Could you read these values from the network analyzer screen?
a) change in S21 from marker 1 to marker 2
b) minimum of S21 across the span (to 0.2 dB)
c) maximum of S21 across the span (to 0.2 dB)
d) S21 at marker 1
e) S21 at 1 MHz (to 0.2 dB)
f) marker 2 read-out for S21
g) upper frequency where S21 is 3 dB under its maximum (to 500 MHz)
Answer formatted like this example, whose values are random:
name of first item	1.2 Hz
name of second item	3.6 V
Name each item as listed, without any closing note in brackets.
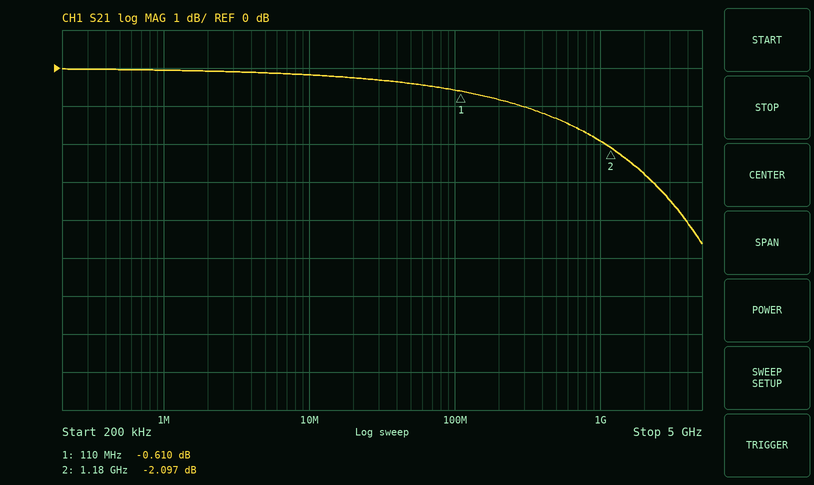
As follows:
change in S21 from marker 1 to marker 2	-1.487 dB
minimum of S21 across the span	-4.6 dB
maximum of S21 across the span	0.0 dB
S21 at marker 1	-0.610 dB
S21 at 1 MHz	0.0 dB
marker 2 read-out for S21	-2.097 dB
upper frequency where S21 is 3 dB under its maximum	2.5 GHz
